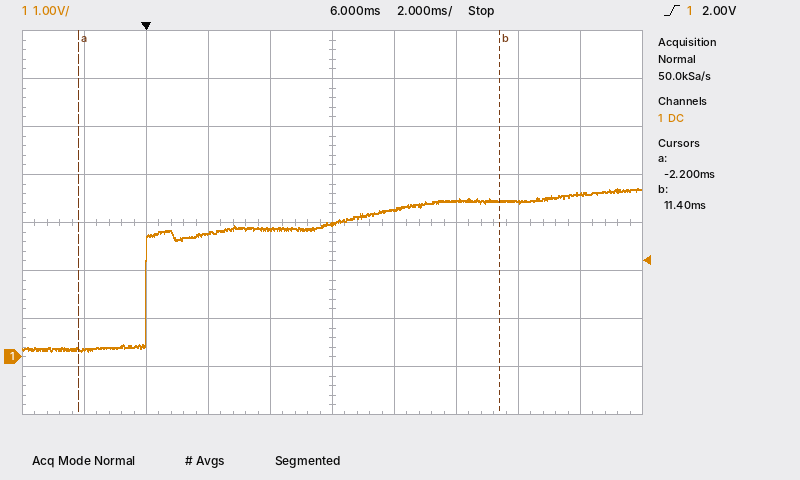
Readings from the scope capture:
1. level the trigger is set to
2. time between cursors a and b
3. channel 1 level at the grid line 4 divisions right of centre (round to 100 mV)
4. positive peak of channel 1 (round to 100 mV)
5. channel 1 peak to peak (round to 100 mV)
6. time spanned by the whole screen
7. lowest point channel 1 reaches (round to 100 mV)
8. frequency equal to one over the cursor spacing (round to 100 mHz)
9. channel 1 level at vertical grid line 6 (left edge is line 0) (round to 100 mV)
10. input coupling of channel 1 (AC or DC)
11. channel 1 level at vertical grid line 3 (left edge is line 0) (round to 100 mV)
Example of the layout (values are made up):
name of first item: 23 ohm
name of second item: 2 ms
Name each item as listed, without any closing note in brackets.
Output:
level the trigger is set to: 2.00 V
time between cursors a and b: 13.6 ms
channel 1 level at the grid line 4 divisions right of centre: 3.4 V
positive peak of channel 1: 3.5 V
channel 1 peak to peak: 3.4 V
time spanned by the whole screen: 20 ms
lowest point channel 1 reaches: 100 mV
frequency equal to one over the cursor spacing: 73.5 Hz
channel 1 level at vertical grid line 6 (left edge is line 0): 3.1 V
input coupling of channel 1: DC
channel 1 level at vertical grid line 3 (left edge is line 0): 2.6 V
